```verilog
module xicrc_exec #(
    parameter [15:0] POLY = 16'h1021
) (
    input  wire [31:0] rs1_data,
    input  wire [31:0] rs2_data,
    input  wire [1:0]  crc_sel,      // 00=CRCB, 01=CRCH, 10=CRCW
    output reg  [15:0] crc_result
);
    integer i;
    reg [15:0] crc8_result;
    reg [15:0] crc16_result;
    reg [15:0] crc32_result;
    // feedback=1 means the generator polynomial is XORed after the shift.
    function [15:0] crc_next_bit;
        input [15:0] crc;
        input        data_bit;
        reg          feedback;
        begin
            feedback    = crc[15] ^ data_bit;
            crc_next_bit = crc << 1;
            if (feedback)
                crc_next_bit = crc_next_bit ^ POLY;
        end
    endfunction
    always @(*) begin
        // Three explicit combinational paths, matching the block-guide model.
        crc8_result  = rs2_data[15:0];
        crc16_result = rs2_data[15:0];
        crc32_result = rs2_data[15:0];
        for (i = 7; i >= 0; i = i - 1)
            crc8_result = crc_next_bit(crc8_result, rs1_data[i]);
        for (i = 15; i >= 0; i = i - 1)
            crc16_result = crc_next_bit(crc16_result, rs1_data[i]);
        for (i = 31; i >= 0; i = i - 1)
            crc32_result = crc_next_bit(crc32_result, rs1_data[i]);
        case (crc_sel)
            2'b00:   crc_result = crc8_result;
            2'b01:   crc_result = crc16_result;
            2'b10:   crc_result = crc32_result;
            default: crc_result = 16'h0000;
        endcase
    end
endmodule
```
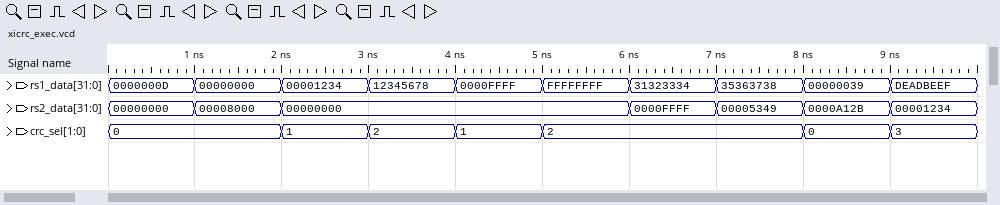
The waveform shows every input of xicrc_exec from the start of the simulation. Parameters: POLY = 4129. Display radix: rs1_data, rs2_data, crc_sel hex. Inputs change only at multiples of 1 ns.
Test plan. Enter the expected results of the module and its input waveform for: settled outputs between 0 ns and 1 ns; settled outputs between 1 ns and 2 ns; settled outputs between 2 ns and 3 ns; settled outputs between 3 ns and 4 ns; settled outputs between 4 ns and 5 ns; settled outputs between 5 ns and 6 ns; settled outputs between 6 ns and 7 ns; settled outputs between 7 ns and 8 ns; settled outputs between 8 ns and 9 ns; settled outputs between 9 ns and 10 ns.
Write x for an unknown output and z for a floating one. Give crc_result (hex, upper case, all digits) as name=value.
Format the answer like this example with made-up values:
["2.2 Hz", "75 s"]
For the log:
["crc_result=D1AD", "crc_result=9188", "crc_result=13C6", "crc_result=B42C", "crc_result=1D0F", "crc_result=99CF", "crc_result=5349", "crc_result=A12B", "crc_result=29B1", "crc_result=0000"]
